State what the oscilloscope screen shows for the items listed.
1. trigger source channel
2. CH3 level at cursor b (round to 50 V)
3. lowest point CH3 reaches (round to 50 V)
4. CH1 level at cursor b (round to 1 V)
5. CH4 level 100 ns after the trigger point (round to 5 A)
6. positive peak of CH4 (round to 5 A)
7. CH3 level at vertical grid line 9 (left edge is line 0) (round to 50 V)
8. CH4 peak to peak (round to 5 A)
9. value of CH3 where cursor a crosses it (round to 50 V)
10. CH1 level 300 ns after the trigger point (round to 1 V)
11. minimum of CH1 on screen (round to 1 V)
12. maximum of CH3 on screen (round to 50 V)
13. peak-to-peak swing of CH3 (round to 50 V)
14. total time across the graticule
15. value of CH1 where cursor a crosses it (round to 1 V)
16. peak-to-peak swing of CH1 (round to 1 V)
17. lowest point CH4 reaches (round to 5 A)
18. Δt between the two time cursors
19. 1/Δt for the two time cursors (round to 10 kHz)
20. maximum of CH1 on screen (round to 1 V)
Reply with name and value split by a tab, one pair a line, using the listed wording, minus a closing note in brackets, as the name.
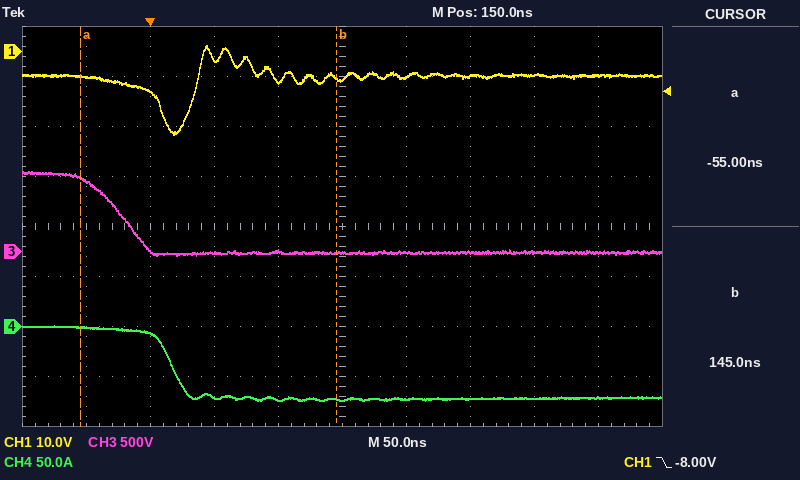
trigger source channel	CH1
CH3 level at cursor b	0 V
lowest point CH3 reaches	-50 V
CH1 level at cursor b	-5 V
CH4 level 100 ns after the trigger point	-75 A
positive peak of CH4	0 A
CH3 level at vertical grid line 9 (left edge is line 0)	0 V
CH4 peak to peak	75 A
value of CH3 where cursor a crosses it	750 V
CH1 level 300 ns after the trigger point	-5 V
minimum of CH1 on screen	-17 V
maximum of CH3 on screen	800 V
peak-to-peak swing of CH3	850 V
total time across the graticule	500 ns
value of CH1 where cursor a crosses it	-5 V
peak-to-peak swing of CH1	18 V
lowest point CH4 reaches	-75 A
Δt between the two time cursors	200 ns
1/Δt for the two time cursors	5.00 MHz
maximum of CH1 on screen	1 V
